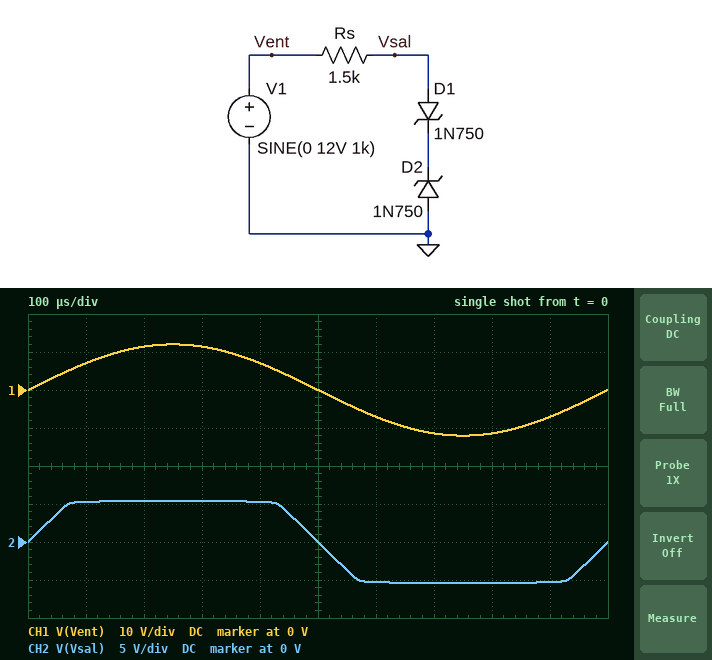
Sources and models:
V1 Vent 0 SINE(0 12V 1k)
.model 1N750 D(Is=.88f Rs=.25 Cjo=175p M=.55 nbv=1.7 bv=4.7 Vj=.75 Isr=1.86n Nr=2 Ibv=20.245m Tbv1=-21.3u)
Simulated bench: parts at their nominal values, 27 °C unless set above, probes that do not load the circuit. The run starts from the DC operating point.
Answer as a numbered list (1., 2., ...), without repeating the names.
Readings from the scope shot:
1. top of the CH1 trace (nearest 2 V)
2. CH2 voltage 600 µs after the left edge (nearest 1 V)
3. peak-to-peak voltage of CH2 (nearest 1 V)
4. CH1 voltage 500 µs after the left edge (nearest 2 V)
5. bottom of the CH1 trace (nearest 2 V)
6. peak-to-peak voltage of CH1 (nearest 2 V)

1. 12 V
2. -5 V
3. 11 V
4. 0 V
5. -12 V
6. 24 V
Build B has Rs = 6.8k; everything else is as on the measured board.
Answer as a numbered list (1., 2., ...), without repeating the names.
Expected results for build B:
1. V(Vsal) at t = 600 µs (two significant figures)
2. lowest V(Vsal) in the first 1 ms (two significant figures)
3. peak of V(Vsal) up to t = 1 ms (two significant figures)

1. -5.2 V
2. -5.3 V
3. 5.3 V
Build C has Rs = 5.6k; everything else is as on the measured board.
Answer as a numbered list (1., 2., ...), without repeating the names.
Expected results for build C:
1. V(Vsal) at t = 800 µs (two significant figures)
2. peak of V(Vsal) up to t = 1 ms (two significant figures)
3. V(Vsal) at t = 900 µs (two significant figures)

1. -5.3 V
2. 5.3 V
3. -5.2 V
